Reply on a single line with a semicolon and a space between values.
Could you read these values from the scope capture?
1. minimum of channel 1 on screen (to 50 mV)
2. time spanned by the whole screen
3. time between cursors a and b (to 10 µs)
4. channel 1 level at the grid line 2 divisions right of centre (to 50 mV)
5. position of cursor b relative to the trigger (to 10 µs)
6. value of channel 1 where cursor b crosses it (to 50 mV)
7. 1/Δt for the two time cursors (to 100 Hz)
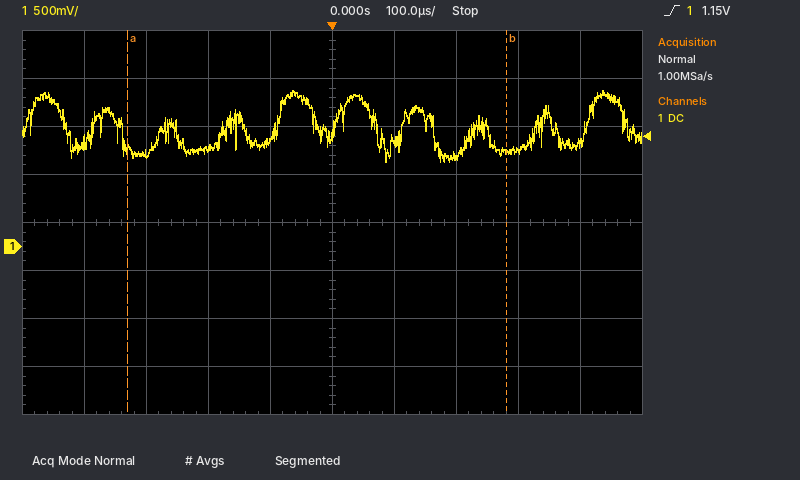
900 mV; 1 ms; 610 µs; 950 mV; +280 µs; 1.00 V; 1.6 kHz
